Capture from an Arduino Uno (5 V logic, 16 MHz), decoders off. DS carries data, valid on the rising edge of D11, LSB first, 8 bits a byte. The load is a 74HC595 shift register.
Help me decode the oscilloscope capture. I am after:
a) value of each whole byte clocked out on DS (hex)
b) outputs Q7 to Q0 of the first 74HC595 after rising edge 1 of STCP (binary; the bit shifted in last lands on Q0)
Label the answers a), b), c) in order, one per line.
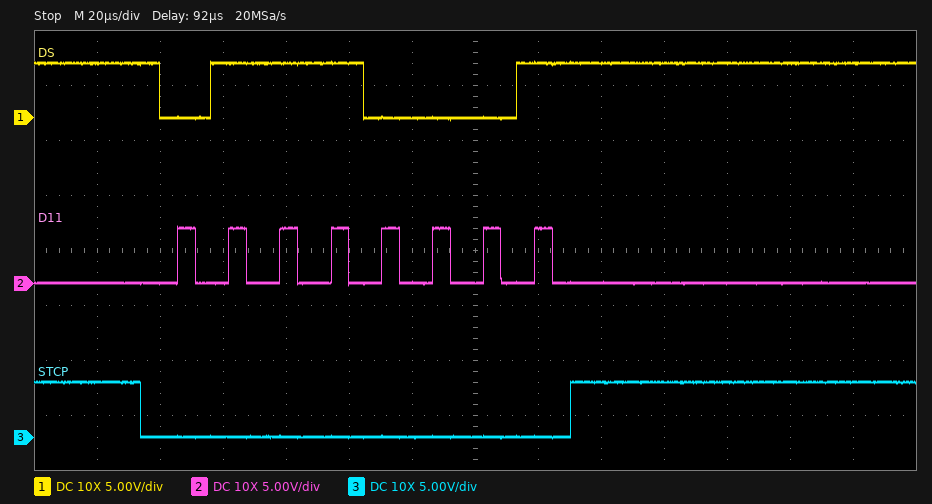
a) 8E
b) 01110001
